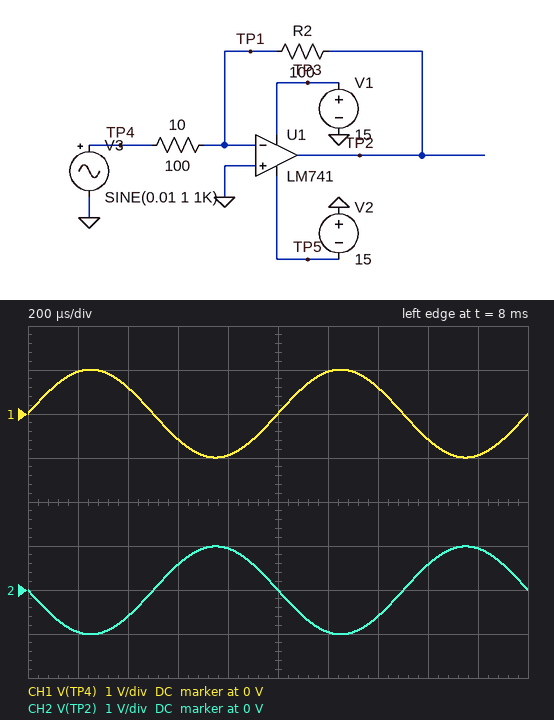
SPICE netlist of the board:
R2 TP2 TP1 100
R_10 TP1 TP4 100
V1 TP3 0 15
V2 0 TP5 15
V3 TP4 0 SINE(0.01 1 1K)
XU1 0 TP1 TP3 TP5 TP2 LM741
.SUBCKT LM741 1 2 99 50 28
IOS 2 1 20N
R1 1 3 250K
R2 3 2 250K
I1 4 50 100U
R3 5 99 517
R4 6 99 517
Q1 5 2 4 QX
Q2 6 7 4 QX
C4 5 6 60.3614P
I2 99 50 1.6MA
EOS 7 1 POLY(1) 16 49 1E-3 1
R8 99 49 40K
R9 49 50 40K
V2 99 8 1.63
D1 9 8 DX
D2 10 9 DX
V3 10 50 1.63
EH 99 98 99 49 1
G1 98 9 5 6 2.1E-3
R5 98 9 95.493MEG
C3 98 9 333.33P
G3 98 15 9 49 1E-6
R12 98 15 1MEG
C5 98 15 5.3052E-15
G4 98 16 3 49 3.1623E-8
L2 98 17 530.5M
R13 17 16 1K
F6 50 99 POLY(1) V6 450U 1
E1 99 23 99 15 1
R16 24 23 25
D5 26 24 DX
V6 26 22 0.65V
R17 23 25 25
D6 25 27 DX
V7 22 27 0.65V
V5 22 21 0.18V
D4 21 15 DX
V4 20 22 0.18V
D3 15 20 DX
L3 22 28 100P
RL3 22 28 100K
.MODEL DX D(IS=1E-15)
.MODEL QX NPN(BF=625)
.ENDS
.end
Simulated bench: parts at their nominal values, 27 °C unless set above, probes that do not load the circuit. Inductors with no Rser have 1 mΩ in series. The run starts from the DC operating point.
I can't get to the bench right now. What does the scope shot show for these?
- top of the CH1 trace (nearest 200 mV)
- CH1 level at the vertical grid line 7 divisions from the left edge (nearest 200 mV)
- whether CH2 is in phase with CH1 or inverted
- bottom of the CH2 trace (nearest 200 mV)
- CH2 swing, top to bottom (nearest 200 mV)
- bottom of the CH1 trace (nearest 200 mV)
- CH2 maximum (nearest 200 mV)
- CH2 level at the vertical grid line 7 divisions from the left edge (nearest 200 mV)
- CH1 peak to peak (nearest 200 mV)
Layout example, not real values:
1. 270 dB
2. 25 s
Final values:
1. 1.0 V
2. 600 mV
3. inverted
4. -1.0 V
5. 2.0 V
6. -1.0 V
7. 1.0 V
8. -600 mV
9. 2.0 V
